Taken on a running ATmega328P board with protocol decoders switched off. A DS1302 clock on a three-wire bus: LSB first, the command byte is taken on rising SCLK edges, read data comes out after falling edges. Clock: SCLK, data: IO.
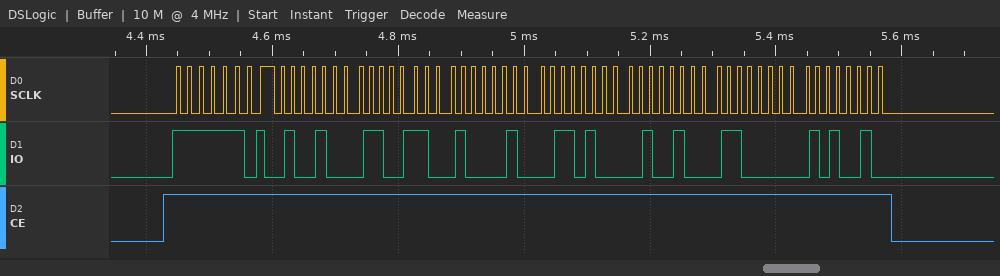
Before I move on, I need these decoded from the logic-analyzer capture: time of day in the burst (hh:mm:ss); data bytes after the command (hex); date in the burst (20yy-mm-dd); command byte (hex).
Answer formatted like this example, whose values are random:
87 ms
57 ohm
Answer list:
21:33:12
12 33 21 16 12 03 25
2025-12-16
0xBF
